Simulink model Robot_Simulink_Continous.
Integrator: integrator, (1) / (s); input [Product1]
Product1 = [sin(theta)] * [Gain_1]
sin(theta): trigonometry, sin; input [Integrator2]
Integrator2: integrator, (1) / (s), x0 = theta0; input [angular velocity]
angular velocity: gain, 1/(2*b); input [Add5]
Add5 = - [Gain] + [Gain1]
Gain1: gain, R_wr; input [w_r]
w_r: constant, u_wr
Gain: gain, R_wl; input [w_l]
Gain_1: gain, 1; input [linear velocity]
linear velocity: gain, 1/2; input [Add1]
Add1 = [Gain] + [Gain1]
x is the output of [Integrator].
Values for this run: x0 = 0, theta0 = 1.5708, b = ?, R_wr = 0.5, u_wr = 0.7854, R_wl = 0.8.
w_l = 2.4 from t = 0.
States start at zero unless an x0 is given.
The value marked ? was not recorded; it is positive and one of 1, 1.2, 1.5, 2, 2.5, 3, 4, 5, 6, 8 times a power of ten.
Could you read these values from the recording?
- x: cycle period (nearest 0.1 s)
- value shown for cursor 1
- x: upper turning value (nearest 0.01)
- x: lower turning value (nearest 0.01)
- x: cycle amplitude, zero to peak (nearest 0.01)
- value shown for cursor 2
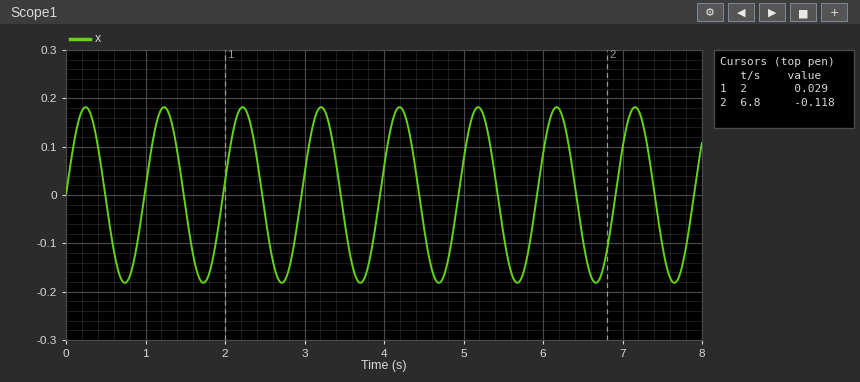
1.0 s
0.029
0.18
-0.18
0.18
-0.118
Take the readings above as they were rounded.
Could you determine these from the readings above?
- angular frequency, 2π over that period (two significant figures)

6.3 rad/s
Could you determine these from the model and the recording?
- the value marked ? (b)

0.12
